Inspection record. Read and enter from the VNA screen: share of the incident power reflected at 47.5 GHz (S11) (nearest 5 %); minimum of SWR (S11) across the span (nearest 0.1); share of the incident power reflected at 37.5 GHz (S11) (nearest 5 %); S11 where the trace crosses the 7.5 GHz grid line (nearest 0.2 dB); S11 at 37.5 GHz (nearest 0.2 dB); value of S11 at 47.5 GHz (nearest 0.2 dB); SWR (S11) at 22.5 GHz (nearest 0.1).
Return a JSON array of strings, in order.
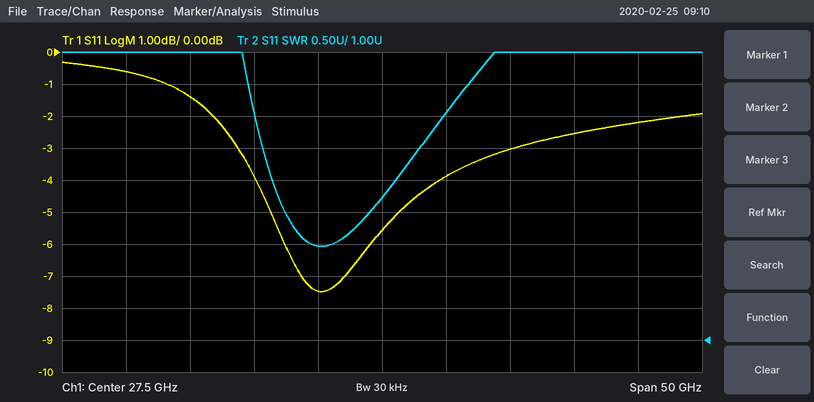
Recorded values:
["60 %", "2.5", "50 %", "-0.6 dB", "-3.0 dB", "-2.2 dB", "2.5"]
